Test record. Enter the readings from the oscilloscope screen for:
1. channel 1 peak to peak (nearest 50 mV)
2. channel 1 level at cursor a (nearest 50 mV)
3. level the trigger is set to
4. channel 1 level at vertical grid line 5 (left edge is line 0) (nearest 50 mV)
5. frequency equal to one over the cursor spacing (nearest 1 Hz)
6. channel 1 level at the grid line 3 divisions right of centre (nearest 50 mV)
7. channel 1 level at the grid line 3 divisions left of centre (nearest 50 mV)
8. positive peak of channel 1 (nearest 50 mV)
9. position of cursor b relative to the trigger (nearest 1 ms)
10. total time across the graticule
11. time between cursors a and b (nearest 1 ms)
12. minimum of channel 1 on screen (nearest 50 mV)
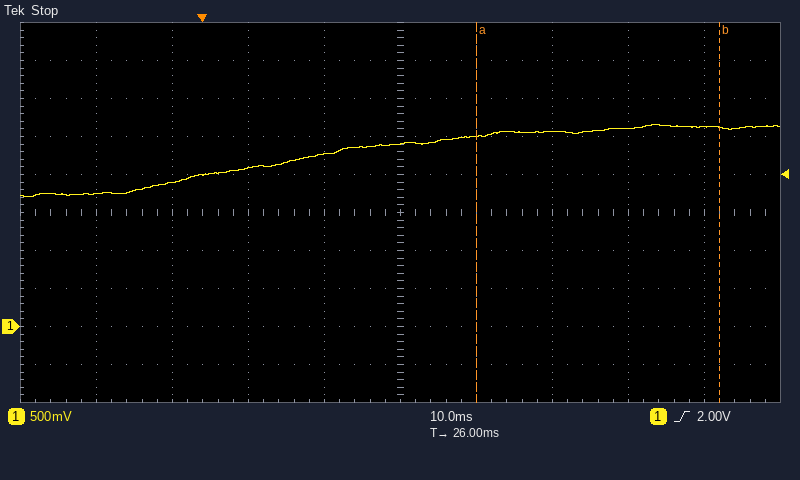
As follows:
950 mV
2.50 V
2.00 V
2.40 V
31 Hz
2.60 V
1.90 V
2.65 V
+68 ms
100 ms
32 ms
1.70 V
